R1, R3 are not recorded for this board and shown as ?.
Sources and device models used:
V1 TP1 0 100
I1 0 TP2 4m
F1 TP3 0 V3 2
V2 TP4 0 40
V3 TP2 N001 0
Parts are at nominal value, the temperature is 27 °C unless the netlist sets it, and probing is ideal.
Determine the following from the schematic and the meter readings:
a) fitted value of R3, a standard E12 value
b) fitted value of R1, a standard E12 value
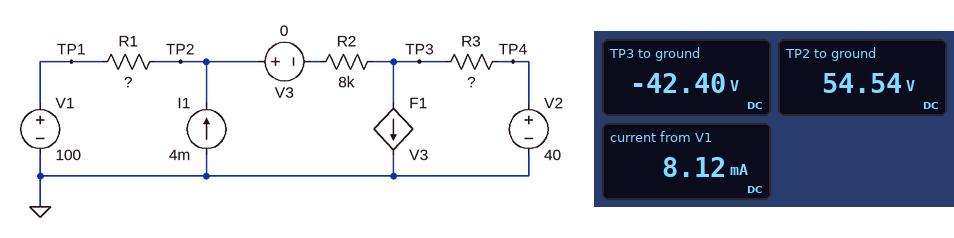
6.8 kΩ
5.6 kΩ
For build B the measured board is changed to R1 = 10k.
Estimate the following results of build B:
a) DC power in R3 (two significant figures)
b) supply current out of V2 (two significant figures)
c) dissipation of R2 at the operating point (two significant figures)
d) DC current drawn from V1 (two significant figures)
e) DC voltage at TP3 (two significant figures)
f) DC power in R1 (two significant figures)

540 mW
8.9 mA
640 mW
4.9 mA
-21 V
240 mW
